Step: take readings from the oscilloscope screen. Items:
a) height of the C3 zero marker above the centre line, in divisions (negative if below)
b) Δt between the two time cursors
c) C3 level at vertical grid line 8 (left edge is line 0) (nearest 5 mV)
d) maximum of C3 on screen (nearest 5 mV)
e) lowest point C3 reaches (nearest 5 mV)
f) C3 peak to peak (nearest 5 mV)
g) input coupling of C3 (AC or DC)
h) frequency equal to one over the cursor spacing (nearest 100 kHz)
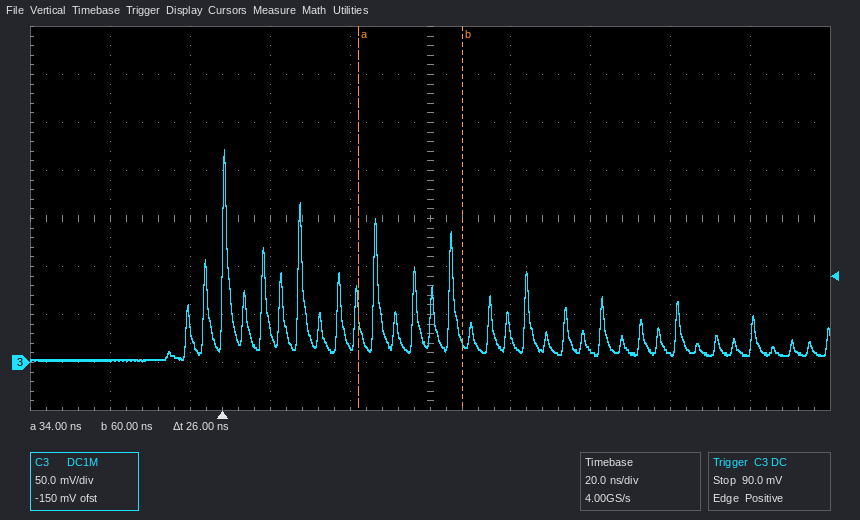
-3.0 div
26 ns
10 mV
220 mV
0 mV
220 mV
DC
38.5 MHz
